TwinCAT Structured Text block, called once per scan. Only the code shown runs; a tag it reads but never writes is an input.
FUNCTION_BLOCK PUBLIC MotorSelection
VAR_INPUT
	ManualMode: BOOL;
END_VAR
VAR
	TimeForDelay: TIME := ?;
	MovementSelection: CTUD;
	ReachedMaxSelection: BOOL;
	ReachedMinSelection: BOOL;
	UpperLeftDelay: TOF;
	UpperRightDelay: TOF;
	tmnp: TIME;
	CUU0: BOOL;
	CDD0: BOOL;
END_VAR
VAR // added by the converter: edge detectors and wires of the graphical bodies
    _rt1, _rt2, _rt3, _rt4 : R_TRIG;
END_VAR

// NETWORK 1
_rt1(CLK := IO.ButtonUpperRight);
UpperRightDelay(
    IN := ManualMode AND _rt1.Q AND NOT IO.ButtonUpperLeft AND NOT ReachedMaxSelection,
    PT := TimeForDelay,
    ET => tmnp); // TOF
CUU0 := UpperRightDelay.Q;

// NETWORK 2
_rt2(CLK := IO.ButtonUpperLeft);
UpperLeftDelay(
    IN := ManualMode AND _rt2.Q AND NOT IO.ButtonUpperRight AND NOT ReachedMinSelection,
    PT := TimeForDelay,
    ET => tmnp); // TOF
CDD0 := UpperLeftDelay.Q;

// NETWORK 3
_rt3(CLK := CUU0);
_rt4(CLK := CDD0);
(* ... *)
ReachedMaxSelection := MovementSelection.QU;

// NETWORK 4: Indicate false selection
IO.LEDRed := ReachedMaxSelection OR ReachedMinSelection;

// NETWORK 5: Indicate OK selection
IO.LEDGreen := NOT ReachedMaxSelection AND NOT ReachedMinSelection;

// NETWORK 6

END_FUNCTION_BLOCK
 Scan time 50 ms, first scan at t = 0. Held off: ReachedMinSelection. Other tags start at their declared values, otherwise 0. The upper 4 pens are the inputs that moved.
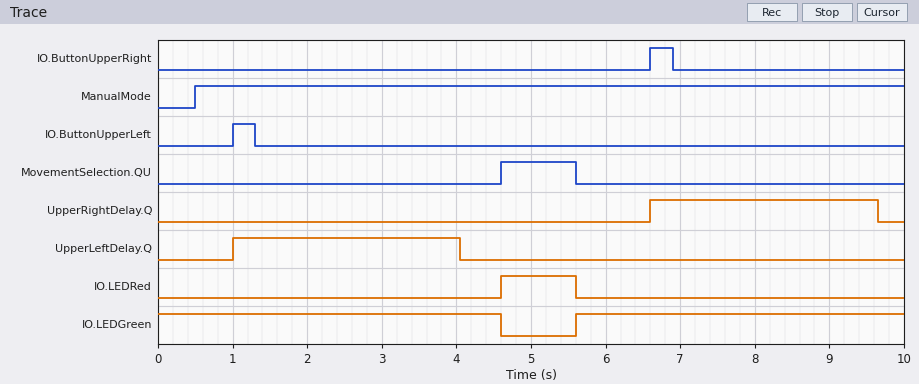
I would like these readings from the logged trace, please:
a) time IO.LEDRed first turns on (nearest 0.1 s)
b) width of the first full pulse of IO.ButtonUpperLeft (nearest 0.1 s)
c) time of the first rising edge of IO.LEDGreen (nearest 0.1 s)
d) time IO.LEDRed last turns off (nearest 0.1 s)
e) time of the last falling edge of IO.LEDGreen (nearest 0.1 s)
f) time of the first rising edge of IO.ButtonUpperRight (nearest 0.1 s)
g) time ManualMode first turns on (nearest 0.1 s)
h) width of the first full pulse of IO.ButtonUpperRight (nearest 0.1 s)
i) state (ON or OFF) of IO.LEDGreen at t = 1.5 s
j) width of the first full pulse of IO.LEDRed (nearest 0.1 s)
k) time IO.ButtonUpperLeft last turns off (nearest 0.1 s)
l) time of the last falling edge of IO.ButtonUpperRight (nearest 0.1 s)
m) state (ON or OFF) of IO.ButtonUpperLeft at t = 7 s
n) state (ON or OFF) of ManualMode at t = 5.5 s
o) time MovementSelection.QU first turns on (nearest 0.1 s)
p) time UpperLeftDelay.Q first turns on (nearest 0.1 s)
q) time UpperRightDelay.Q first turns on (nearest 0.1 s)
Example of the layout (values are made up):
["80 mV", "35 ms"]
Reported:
["4.6 s", "0.3 s", "5.6 s", "5.6 s", "4.6 s", "6.6 s", "0.5 s", "0.3 s", "ON", "1.0 s", "1.3 s", "6.9 s", "OFF", "ON", "4.6 s", "1.0 s", "6.6 s"]
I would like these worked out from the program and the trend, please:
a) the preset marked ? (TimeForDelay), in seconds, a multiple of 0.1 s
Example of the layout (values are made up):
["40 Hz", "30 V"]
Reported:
["3.0 s"]
